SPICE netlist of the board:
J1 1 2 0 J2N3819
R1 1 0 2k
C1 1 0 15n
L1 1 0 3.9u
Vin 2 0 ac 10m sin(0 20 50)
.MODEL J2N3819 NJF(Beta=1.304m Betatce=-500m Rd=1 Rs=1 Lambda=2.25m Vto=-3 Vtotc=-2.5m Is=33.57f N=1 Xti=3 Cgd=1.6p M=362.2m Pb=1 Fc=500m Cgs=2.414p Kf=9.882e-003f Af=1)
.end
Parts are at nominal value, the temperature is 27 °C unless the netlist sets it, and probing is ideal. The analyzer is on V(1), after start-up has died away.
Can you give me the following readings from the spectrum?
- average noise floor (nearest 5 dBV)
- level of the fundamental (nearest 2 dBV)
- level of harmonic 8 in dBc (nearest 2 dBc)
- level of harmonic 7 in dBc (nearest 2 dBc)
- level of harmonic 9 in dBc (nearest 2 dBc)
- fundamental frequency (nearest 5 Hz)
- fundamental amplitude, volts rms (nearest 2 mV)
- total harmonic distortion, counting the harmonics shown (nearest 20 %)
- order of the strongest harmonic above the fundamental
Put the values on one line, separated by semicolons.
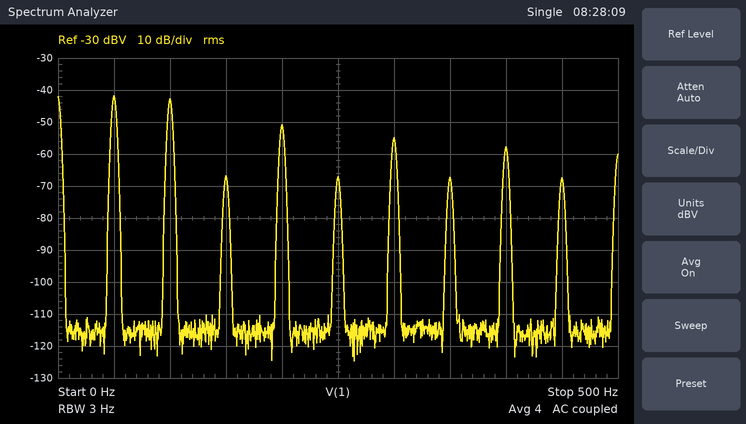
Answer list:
-115 dBV; -42 dBV; -16 dBc; -26 dBc; -26 dBc; 50 Hz; 8 mV; 100 %; 2
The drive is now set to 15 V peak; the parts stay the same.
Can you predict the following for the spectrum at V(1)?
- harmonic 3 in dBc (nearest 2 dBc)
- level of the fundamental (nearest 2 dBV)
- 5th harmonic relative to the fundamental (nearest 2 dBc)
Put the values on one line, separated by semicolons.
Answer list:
-22 dBc; -44 dBV; -22 dBc
